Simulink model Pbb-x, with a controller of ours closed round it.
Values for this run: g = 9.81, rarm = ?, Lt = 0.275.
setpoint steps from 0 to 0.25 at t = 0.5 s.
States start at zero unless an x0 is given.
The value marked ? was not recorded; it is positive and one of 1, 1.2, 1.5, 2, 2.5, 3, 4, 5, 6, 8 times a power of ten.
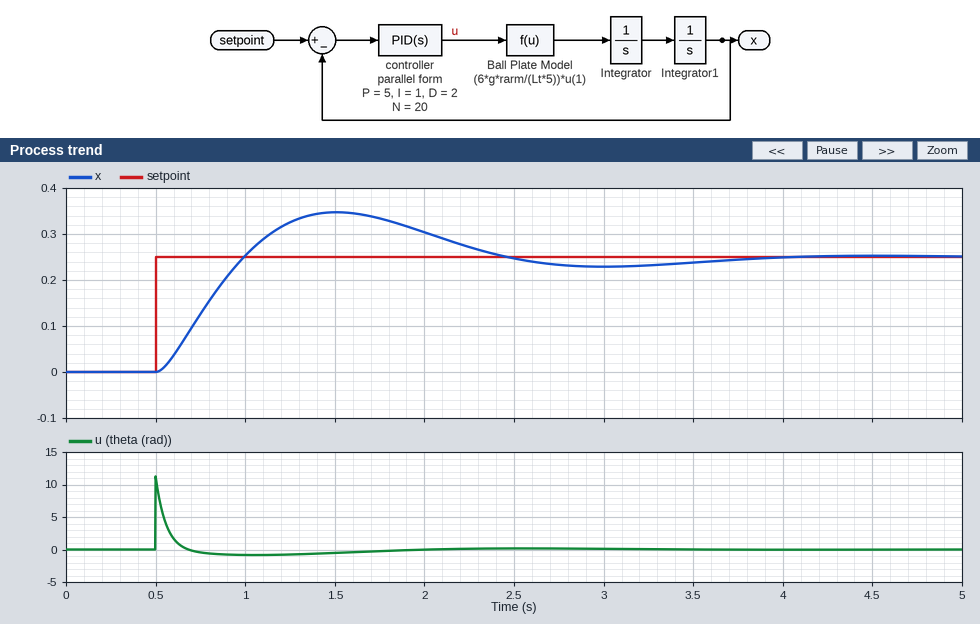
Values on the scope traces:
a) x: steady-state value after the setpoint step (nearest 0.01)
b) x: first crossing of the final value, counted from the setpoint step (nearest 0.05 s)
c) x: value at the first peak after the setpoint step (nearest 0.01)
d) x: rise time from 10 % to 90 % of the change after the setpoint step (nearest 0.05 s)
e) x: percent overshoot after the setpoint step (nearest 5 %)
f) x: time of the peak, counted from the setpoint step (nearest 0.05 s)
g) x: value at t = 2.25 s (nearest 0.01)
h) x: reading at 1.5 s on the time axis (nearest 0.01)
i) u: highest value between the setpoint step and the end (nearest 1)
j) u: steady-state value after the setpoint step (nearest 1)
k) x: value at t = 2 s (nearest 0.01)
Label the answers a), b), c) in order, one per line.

a) 0.25
b) 0.50 s
c) 0.35
d) 0.35 s
e) 40 %
f) 1.00 s
g) 0.27
h) 0.35
i) 11
j) 0
k) 0.30
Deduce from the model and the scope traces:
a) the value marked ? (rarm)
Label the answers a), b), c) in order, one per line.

a) 0.025
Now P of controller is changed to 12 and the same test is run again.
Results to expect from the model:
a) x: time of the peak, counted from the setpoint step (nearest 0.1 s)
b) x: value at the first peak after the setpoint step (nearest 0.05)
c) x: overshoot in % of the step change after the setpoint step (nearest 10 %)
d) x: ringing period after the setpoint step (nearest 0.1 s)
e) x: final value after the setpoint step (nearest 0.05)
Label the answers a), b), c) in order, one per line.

a) 0.7 s
b) 0.40
c) 50 %
d) 1.7 s
e) 0.25
